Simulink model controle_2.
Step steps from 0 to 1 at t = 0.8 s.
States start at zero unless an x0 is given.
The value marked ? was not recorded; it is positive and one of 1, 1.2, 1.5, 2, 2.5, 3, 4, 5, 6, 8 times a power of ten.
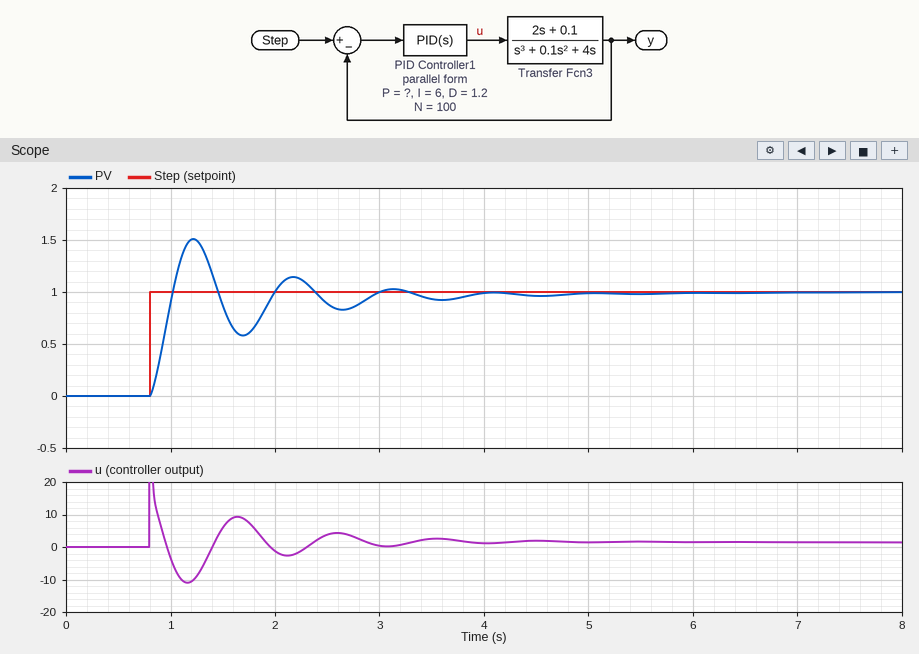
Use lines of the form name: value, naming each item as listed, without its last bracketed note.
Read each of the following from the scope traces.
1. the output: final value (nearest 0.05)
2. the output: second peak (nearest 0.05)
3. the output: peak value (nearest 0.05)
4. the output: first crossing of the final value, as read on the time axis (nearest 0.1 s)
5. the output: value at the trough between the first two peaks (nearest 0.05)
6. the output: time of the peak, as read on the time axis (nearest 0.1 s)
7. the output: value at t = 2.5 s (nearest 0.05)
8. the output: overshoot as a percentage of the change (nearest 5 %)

the output: final value: 1.00
the output: second peak: 1.15
the output: peak value: 1.50
the output: first crossing of the final value, as read on the time axis: 1.0 s
the output: value at the trough between the first two peaks: 0.60
the output: time of the peak, as read on the time axis: 1.2 s
the output: value at t = 2.5 s: 0.90
the output: overshoot as a percentage of the change: 50 %
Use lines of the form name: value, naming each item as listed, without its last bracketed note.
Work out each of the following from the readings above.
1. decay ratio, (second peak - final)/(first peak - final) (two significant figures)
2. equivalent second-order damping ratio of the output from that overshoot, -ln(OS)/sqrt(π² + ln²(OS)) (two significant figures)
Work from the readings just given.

decay ratio, (second peak - final)/(first peak - final): 0.30
equivalent second-order damping ratio of the output from that overshoot, -ln(OS)/sqrt(π² + ln²(OS)): 0.22
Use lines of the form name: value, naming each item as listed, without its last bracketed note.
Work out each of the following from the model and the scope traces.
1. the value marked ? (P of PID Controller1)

the value marked ?: 20
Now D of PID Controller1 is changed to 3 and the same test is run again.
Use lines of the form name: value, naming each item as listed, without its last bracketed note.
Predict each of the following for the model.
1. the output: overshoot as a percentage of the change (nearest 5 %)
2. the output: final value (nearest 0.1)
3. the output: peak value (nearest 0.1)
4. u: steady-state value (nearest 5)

the output: overshoot as a percentage of the change: 25 %
the output: final value: 1.0
the output: peak value: 1.3
u: steady-state value: 0
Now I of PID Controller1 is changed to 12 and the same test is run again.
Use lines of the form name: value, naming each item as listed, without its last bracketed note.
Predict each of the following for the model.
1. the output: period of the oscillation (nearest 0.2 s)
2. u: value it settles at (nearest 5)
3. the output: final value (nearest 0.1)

the output: period of the oscillation: 1.0 s
u: value it settles at: 0
the output: final value: 1.0
